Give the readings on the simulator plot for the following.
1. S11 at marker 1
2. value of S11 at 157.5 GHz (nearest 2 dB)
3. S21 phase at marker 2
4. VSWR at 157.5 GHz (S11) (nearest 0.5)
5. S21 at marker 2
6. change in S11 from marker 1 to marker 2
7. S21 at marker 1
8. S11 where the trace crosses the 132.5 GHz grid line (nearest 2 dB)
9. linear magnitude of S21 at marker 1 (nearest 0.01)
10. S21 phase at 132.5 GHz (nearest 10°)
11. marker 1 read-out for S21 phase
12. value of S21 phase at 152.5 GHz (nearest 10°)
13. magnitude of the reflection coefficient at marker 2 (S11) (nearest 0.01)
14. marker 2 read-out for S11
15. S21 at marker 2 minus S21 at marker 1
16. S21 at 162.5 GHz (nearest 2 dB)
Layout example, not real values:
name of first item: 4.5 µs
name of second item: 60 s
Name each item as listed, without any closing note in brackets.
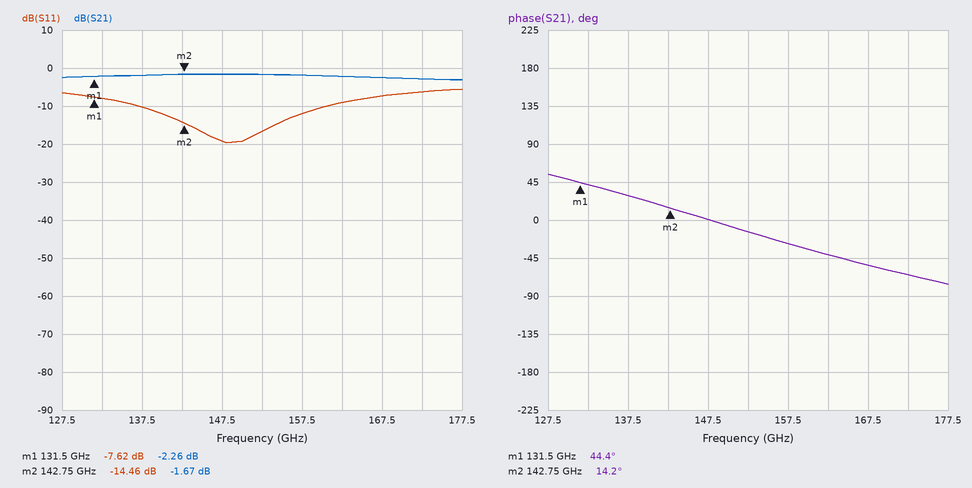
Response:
S11 at marker 1: -7.62 dB
value of S11 at 157.5 GHz: -12 dB
S21 phase at marker 2: 14.2°
VSWR at 157.5 GHz (S11): 1.5
S21 at marker 2: -1.67 dB
change in S11 from marker 1 to marker 2: -6.84 dB
S21 at marker 1: -2.26 dB
S11 where the trace crosses the 132.5 GHz grid line: -8 dB
linear magnitude of S21 at marker 1: 0.77
S21 phase at 132.5 GHz: 40°
marker 1 read-out for S21 phase: 44.4°
value of S21 phase at 152.5 GHz: -10°
magnitude of the reflection coefficient at marker 2 (S11): 0.19
marker 2 read-out for S11: -14.46 dB
S21 at marker 2 minus S21 at marker 1: 0.59 dB
S21 at 162.5 GHz: -2 dB
